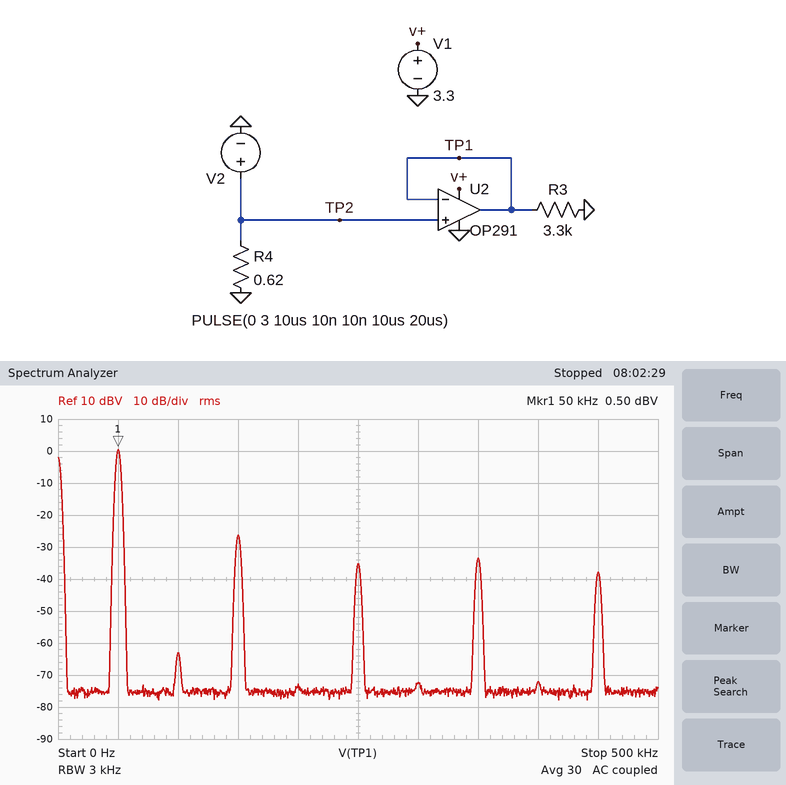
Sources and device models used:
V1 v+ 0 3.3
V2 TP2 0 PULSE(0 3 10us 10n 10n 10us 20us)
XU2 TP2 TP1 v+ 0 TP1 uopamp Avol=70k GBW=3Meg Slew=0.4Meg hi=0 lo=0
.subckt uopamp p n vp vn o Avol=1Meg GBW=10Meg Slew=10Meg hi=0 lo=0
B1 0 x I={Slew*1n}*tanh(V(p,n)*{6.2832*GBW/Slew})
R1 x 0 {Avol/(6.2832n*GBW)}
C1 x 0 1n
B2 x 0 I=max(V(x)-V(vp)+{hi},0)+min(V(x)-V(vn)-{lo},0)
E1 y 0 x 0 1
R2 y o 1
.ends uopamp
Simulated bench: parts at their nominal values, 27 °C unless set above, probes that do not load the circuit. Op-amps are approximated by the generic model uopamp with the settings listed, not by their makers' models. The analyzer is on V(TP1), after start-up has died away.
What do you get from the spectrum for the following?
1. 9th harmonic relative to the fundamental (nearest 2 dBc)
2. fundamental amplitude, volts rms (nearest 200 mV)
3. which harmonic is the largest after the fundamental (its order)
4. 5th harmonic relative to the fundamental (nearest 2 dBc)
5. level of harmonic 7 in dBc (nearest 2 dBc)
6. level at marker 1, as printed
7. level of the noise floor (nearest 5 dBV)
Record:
-38 dBc
1.0 V
3
-36 dBc
-34 dBc
0.50 dBV
-75 dBV
